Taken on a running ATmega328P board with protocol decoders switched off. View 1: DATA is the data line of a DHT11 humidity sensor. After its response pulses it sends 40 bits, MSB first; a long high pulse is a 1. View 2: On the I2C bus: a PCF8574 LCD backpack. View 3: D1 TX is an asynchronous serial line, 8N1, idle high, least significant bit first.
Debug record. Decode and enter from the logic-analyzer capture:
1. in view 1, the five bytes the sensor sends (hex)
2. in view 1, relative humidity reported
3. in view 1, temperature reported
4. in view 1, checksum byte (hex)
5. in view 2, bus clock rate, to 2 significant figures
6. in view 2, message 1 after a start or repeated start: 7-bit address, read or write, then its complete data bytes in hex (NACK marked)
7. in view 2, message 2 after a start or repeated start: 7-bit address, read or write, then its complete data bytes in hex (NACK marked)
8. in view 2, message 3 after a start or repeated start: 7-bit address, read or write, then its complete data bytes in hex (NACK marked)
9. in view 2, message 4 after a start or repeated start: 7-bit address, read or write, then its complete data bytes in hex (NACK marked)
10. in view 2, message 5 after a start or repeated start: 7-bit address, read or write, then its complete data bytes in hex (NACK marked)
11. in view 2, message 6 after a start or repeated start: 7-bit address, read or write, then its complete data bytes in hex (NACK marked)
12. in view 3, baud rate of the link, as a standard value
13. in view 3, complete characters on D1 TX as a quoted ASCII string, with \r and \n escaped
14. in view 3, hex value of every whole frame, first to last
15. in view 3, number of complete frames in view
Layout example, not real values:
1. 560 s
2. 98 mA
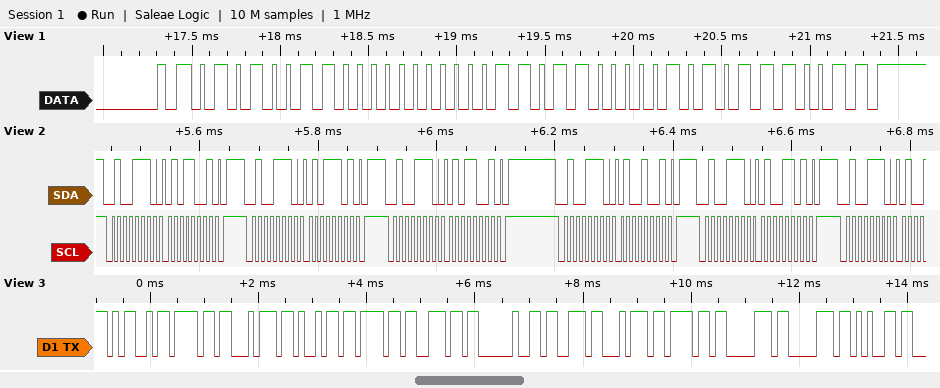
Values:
1. 53 00 1B 05 73
2. 83 %
3. 27.5 °C
4. 0x73
5. 100 kHz
6. 0x27 write: 59
7. 0x27 write: 5D
8. 0x27 write: 59
9. 0x27 write: 49
10. 0x27 write: 4D
11. 0x27 write
12. 9600 baud
13. "Motion stoppe"
14. 4D 6F 74 69 6F 6E 20 73 74 6F 70 70 65
15. 13
